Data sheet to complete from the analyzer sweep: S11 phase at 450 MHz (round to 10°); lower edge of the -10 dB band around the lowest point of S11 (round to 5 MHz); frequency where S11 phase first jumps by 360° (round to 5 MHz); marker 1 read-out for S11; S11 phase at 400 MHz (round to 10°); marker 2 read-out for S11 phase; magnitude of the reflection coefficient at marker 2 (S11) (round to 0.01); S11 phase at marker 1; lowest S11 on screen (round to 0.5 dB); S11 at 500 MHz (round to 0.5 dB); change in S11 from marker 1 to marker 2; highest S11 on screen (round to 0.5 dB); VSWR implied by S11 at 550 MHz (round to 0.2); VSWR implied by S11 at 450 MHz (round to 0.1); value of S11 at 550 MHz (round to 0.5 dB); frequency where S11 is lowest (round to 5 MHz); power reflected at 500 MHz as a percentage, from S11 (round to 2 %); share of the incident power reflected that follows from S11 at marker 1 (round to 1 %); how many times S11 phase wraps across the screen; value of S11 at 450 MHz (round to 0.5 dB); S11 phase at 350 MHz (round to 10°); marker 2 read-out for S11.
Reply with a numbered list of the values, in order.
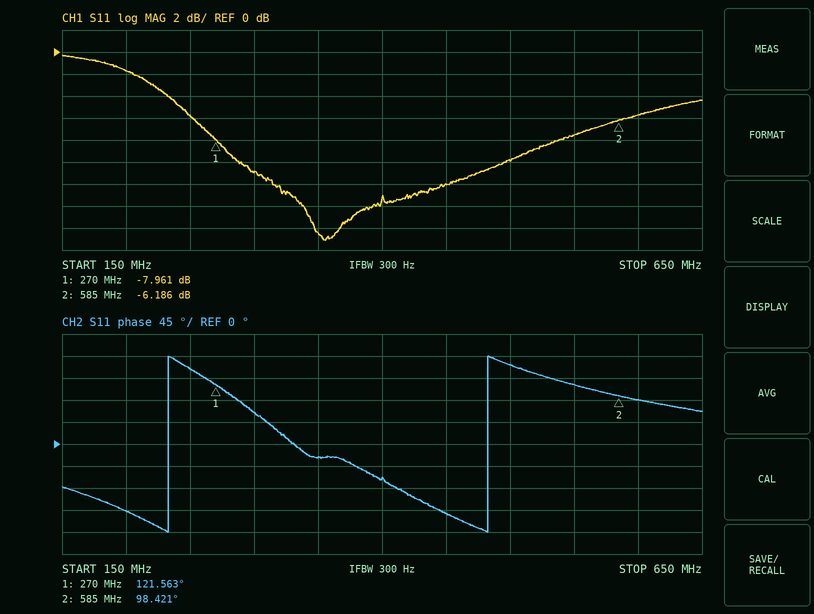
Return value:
1. -140°
2. 290 MHz
3. 235 MHz
4. -7.961 dB
5. -70°
6. 98.421°
7. 0.49
8. 121.563°
9. -17.0 dB
10. -10.0 dB
11. 1.775 dB
12. -0.5 dB
13. 2.4
14. 1.7
15. -7.5 dB
16. 355 MHz
17. 10 %
18. 16 %
19. 2
20. -12.0 dB
21. -30°
22. -6.186 dB
